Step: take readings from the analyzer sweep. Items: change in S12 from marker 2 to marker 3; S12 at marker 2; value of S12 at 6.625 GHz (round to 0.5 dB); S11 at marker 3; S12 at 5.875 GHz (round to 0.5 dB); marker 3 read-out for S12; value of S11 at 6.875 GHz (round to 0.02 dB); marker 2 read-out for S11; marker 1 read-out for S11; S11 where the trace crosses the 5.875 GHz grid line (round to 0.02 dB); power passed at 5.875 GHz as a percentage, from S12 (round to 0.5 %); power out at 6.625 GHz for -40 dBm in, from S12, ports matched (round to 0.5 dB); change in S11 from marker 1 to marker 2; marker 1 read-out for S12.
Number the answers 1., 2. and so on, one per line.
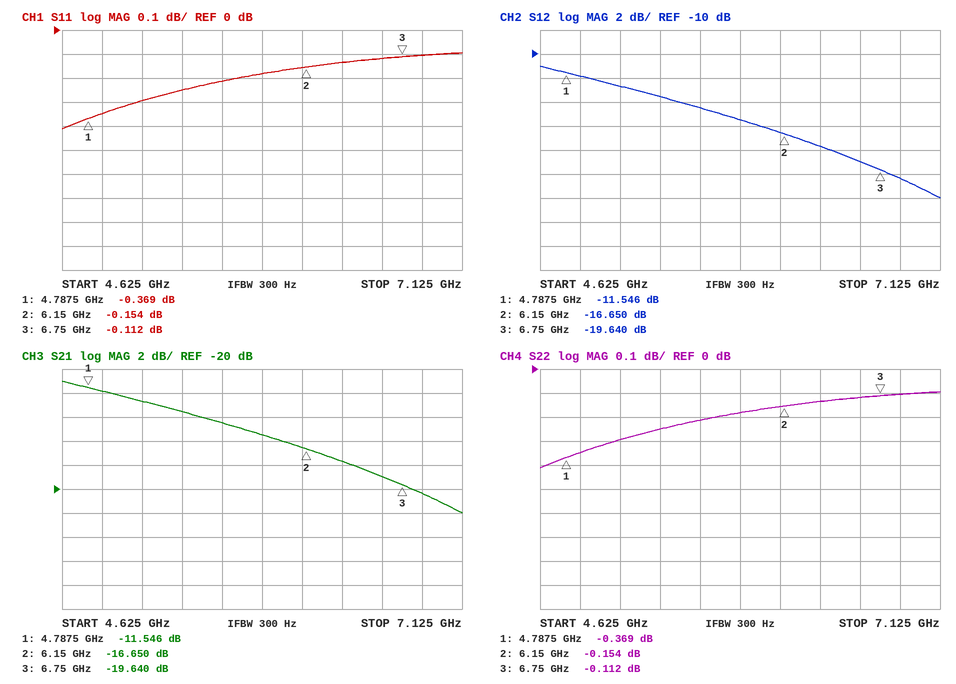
1. -2.990 dB
2. -16.650 dB
3. -19.0 dB
4. -0.112 dB
5. -15.5 dB
6. -19.640 dB
7. -0.10 dB
8. -0.154 dB
9. -0.369 dB
10. -0.18 dB
11. 3.0 %
12. -59.0 dBm
13. 0.215 dB
14. -11.546 dB
